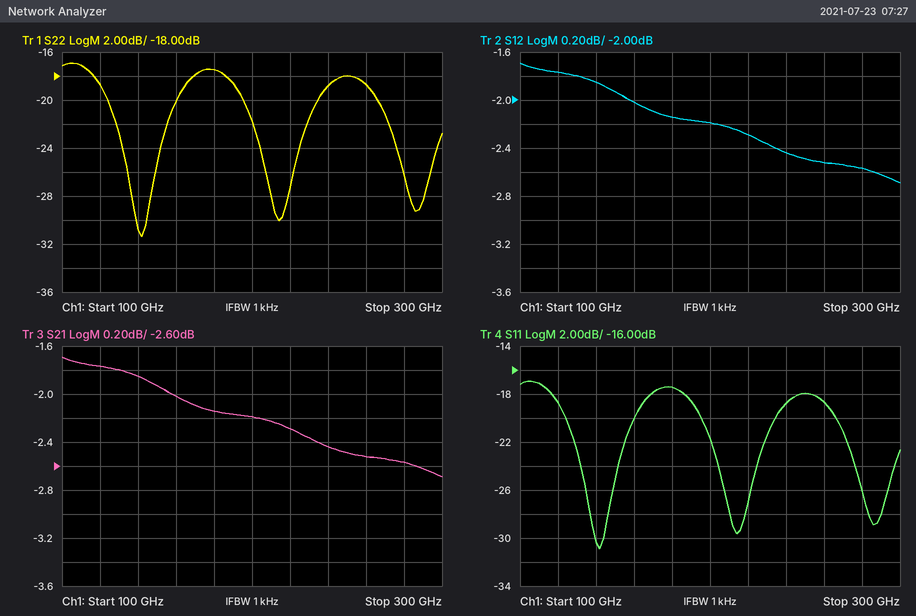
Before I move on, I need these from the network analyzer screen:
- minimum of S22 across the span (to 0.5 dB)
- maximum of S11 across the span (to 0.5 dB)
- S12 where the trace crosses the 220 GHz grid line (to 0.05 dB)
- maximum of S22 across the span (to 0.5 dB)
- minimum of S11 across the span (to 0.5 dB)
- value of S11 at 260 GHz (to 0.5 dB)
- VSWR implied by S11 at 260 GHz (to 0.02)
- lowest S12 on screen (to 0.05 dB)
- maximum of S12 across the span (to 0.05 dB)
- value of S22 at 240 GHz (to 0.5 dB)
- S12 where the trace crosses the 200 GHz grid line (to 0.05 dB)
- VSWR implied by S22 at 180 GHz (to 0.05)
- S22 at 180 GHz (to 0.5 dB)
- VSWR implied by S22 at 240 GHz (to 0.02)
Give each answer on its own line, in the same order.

-31.5 dB
-17.0 dB
-2.30 dB
-17.0 dB
-31.0 dB
-18.5 dB
1.26
-2.70 dB
-1.70 dB
-19.0 dB
-2.20 dB
1.30
-17.5 dB
1.26
